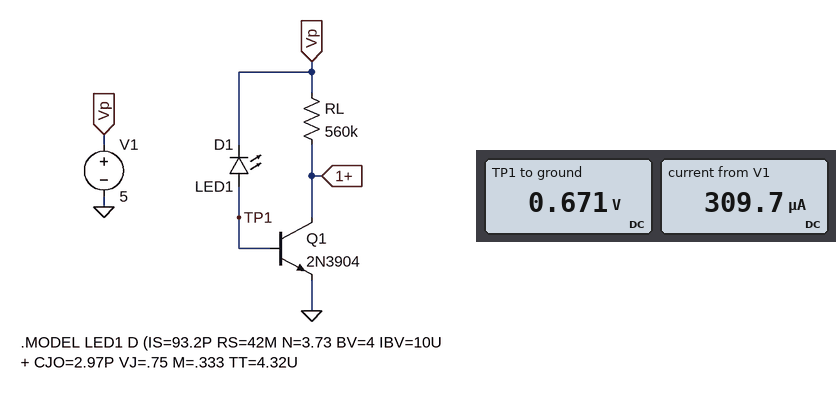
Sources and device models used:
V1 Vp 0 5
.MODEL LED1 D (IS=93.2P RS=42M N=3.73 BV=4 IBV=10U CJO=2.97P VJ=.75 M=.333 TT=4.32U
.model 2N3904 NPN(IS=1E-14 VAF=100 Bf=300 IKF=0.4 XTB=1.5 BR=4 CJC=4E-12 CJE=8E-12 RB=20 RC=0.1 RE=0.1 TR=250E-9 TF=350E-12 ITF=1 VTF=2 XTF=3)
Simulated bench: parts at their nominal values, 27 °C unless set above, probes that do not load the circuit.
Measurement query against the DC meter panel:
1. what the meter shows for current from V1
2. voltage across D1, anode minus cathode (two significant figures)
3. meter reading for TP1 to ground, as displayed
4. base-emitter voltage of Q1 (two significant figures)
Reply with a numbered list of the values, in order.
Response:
1. 309.7 µA
2. -4.3 V
3. 0.671 V
4. 670 mV
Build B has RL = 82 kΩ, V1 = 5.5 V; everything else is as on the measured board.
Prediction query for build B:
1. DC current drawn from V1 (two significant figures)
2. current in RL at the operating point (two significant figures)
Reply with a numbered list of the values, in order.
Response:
1. 6.5 mA
2. 67 µA
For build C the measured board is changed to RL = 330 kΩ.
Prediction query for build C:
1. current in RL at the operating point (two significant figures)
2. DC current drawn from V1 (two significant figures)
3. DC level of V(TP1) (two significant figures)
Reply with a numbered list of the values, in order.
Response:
1. 15 µA
2. 320 µA
3. 670 mV
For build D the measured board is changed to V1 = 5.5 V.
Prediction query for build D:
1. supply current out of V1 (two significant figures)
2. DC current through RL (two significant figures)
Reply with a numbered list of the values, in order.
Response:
1. 6.5 mA
2. 9.8 µA
